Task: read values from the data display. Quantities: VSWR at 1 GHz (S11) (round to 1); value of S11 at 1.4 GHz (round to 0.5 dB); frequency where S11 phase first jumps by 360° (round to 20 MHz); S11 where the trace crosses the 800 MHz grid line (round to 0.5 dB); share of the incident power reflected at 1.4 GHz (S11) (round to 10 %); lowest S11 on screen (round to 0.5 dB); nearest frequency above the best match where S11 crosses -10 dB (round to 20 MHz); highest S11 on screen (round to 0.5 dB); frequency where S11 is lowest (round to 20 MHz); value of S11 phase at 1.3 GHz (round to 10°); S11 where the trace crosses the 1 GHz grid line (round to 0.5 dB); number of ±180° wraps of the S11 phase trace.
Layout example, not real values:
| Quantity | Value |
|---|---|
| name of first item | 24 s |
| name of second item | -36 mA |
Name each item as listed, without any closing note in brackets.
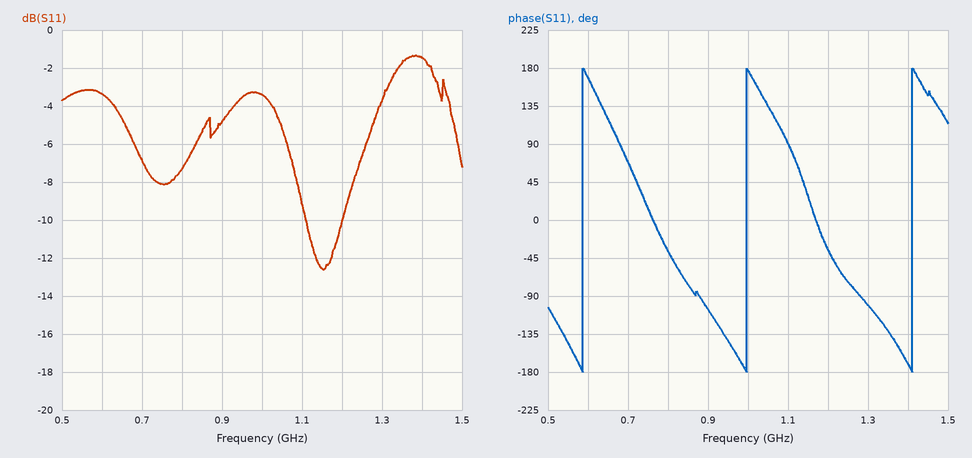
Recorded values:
| Quantity | Value |
|---|---|
| VSWR at 1 GHz (S11) | 5 |
| value of S11 at 1.4 GHz | -1.5 dB |
| frequency where S11 phase first jumps by 360° | 580 MHz |
| S11 where the trace crosses the 800 MHz grid line | -7.5 dB |
| share of the incident power reflected at 1.4 GHz (S11) | 70 % |
| lowest S11 on screen | -12.5 dB |
| nearest frequency above the best match where S11 crosses -10 dB | 1.20 GHz |
| highest S11 on screen | -1.5 dB |
| frequency where S11 is lowest | 1.16 GHz |
| value of S11 phase at 1.3 GHz | -100° |
| S11 where the trace crosses the 1 GHz grid line | -3.5 dB |
| number of ±180° wraps of the S11 phase trace | 3 |
